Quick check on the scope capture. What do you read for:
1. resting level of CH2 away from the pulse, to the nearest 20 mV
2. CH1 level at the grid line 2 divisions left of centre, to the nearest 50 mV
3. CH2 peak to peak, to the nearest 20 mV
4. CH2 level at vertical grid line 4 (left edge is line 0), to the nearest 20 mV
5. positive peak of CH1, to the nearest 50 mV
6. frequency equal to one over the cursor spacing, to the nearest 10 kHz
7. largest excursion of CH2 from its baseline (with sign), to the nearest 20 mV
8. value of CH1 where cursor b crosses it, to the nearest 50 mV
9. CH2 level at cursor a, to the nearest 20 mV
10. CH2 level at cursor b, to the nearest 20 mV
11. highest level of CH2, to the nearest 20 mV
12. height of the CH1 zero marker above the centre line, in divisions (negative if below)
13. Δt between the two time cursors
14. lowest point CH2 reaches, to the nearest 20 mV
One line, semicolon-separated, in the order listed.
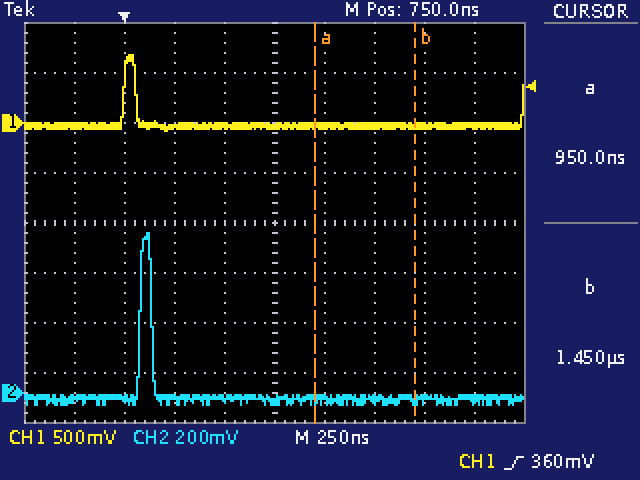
-20 mV; -50 mV; 680 mV; -20 mV; 700 mV; 2.00 MHz; +660 mV; -50 mV; -20 mV; -20 mV; 640 mV; +2.0 div; 500 ns; -40 mV
